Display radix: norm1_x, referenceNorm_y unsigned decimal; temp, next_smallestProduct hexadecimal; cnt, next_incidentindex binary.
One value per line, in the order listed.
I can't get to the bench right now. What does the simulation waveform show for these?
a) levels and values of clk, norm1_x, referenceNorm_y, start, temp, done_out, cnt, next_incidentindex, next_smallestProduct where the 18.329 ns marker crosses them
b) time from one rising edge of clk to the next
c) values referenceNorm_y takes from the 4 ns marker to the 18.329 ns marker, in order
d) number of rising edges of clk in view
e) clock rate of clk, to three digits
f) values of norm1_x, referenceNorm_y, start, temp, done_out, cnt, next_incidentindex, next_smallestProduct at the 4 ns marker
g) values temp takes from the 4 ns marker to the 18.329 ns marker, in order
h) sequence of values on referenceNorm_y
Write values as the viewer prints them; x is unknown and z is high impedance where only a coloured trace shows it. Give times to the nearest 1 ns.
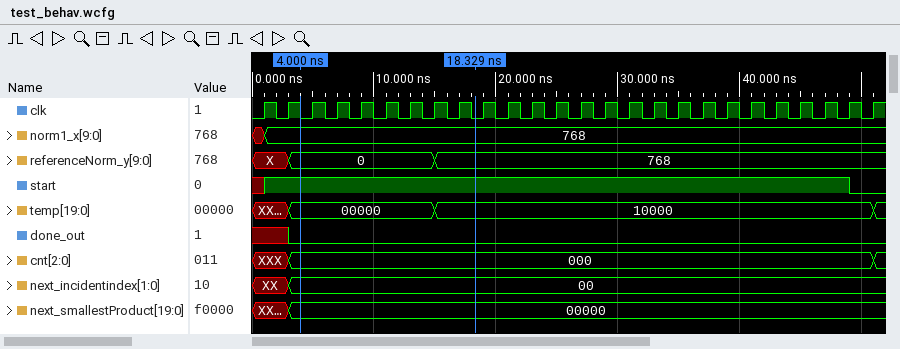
clk=0, norm1_x=768, referenceNorm_y=768, start=1, temp=10000, done_out=0, cnt=000, next_incidentindex=00, next_smallestProduct=00000
2 ns
0, 768
26
500 MHz
norm1_x=768, referenceNorm_y=0, start=1, temp=00000, done_out=0, cnt=000, next_incidentindex=00, next_smallestProduct=00000
00000, 10000
X, 0, 768
